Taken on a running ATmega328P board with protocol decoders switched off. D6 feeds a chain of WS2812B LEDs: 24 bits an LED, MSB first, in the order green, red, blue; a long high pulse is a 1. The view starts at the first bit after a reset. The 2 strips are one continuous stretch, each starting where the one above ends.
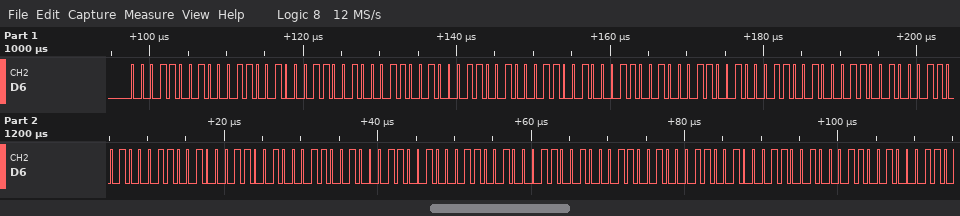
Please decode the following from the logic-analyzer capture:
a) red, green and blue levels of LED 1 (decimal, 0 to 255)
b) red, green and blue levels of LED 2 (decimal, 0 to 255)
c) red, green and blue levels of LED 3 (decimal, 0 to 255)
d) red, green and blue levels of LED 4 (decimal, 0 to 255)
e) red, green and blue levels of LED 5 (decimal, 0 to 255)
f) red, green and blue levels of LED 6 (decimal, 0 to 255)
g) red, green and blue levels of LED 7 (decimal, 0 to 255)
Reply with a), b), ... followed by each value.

a) 25, 25, 25
b) 25, 25, 25
c) 25, 25, 25
d) 25, 25, 25
e) 25, 25, 25
f) 25, 25, 25
g) 25, 25, 25
